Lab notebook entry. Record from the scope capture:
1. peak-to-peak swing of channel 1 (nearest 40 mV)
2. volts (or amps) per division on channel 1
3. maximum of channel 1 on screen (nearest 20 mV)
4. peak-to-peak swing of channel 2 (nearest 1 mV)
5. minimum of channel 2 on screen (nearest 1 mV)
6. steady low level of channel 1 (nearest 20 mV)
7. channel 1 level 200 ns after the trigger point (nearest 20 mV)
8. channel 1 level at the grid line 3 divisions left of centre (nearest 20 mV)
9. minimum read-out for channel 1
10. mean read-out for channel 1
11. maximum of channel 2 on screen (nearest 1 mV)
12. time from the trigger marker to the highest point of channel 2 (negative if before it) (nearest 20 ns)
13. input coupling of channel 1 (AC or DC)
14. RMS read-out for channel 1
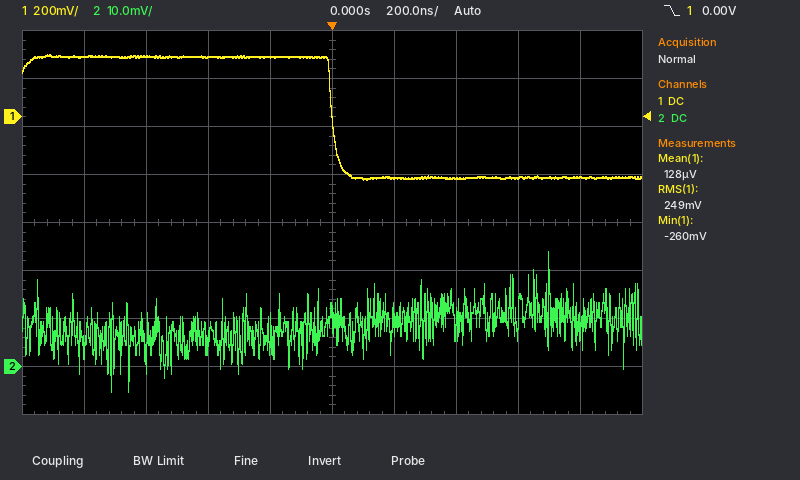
520 mV
200 mV
260 mV
29 mV
-5 mV
-260 mV
-260 mV
260 mV
-260 mV
128 µV
24 mV
+700 ns
DC
249 mV
